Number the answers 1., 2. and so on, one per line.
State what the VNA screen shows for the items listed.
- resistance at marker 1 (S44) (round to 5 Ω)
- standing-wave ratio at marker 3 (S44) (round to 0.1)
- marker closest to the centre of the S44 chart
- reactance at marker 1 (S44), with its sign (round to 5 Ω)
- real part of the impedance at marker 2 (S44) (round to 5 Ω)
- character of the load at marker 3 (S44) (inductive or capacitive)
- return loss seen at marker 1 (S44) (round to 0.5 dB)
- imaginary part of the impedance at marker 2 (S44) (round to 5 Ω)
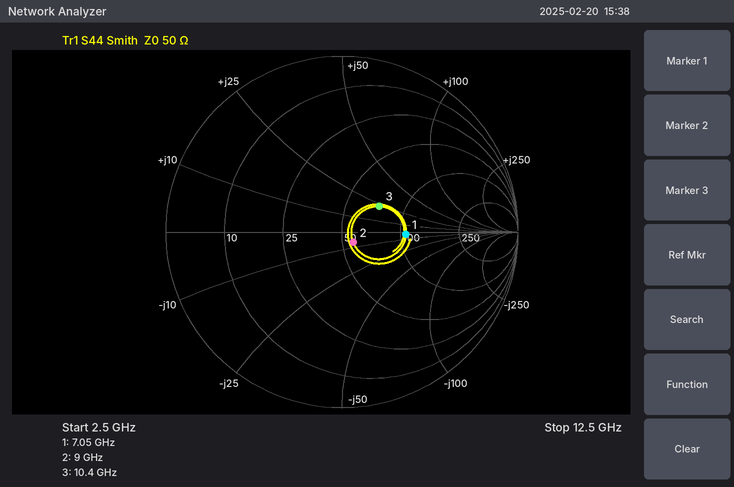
1. 105 Ω
2. 1.7
3. marker 2
4. -5 Ω
5. 55 Ω
6. inductive
7. 9.0 dB
8. -5 Ω
